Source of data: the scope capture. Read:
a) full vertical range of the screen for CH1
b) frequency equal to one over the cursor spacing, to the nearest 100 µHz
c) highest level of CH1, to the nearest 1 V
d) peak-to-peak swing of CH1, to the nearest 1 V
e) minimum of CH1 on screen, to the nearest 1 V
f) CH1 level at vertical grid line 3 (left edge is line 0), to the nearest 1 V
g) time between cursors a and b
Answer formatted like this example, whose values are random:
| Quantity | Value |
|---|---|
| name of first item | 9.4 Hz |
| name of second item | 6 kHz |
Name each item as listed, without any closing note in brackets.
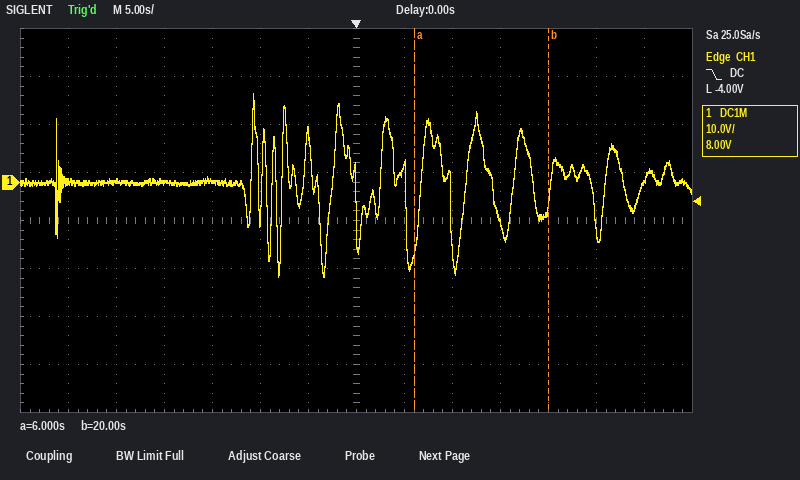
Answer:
| Quantity | Value |
|---|---|
| full vertical range of the screen for CH1 | 80 V |
| frequency equal to one over the cursor spacing, to the nearest 100 µHz | 71.4 mHz |
| highest level of CH1, to the nearest 1 V | 18 V |
| peak-to-peak swing of CH1, to the nearest 1 V | 38 V |
| minimum of CH1 on screen, to the nearest 1 V | -20 V |
| CH1 level at vertical grid line 3 (left edge is line 0), to the nearest 1 V | 0 V |
| time between cursors a and b | 14.0 s |
